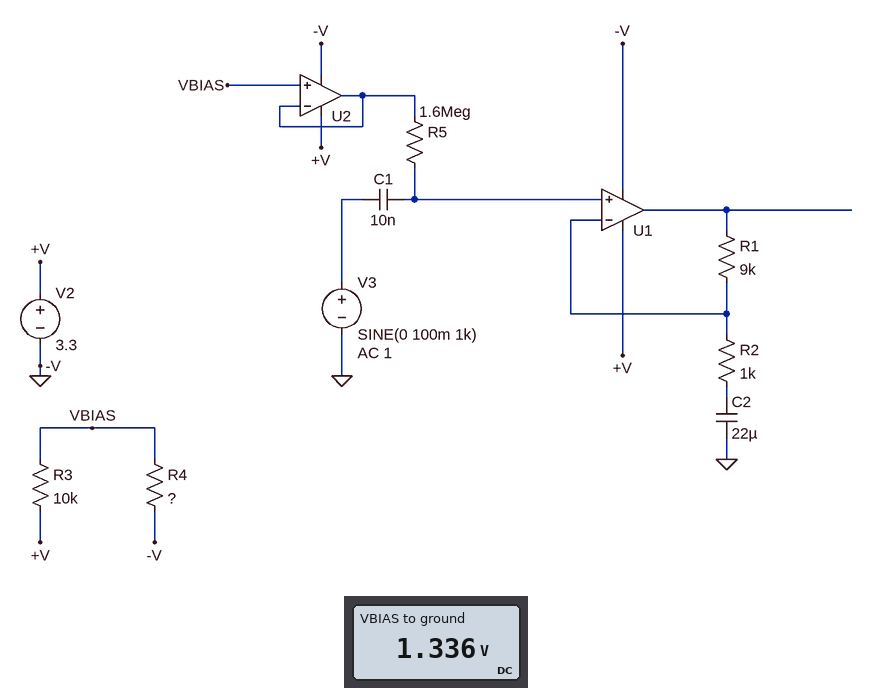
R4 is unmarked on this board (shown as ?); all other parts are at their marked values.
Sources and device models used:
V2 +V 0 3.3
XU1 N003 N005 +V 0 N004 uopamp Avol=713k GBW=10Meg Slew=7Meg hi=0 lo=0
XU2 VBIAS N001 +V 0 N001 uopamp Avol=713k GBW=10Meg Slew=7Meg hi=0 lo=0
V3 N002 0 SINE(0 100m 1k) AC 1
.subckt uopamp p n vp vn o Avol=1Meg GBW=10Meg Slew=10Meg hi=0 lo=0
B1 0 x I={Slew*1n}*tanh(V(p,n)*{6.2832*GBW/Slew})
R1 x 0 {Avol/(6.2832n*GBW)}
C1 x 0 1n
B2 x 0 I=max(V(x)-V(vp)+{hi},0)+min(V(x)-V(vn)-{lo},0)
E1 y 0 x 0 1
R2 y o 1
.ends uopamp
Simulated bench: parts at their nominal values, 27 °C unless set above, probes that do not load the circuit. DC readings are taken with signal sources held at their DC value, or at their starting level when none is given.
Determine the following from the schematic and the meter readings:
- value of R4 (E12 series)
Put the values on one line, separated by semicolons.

6.8 kΩ
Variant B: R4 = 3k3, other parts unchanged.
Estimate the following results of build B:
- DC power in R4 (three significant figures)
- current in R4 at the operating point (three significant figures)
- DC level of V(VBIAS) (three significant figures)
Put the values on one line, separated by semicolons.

203 µW; 248 µA; 819 mV
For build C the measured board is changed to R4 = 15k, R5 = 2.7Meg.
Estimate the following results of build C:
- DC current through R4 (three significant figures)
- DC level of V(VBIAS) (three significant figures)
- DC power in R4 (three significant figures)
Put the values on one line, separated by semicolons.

132 µA; 1.98 V; 261 µW
